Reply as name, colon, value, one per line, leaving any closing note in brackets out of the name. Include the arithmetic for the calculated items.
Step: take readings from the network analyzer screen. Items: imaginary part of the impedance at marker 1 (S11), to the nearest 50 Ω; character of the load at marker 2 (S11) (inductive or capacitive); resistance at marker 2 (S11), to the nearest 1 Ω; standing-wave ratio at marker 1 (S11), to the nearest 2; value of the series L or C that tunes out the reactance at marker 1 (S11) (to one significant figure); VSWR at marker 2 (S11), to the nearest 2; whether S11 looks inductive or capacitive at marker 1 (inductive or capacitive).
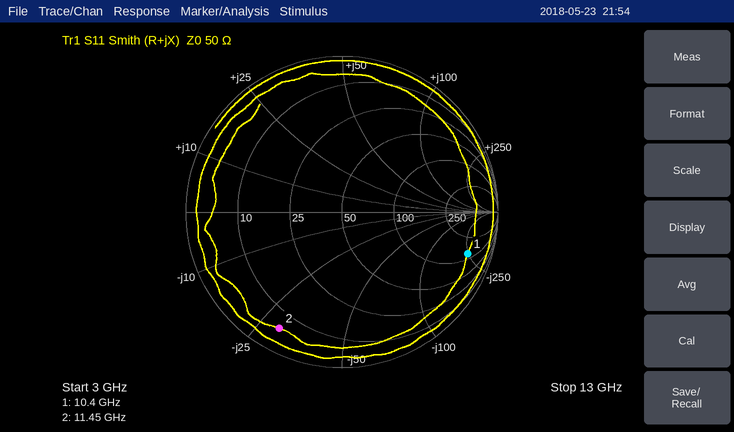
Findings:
imaginary part of the impedance at marker 1 (S11), to the nearest 50 Ω: -250 Ω
character of the load at marker 2 (S11): capacitive
resistance at marker 2 (S11), to the nearest 1 Ω: 6 Ω
standing-wave ratio at marker 1 (S11), to the nearest 2: 12
value of the series L or C that tunes out the reactance at marker 1 (S11): L = 250 Ω/(2π × 10.4 GHz) ≈ 4 nH
VSWR at marker 2 (S11), to the nearest 2: 12
whether S11 looks inductive or capacitive at marker 1: capacitive
